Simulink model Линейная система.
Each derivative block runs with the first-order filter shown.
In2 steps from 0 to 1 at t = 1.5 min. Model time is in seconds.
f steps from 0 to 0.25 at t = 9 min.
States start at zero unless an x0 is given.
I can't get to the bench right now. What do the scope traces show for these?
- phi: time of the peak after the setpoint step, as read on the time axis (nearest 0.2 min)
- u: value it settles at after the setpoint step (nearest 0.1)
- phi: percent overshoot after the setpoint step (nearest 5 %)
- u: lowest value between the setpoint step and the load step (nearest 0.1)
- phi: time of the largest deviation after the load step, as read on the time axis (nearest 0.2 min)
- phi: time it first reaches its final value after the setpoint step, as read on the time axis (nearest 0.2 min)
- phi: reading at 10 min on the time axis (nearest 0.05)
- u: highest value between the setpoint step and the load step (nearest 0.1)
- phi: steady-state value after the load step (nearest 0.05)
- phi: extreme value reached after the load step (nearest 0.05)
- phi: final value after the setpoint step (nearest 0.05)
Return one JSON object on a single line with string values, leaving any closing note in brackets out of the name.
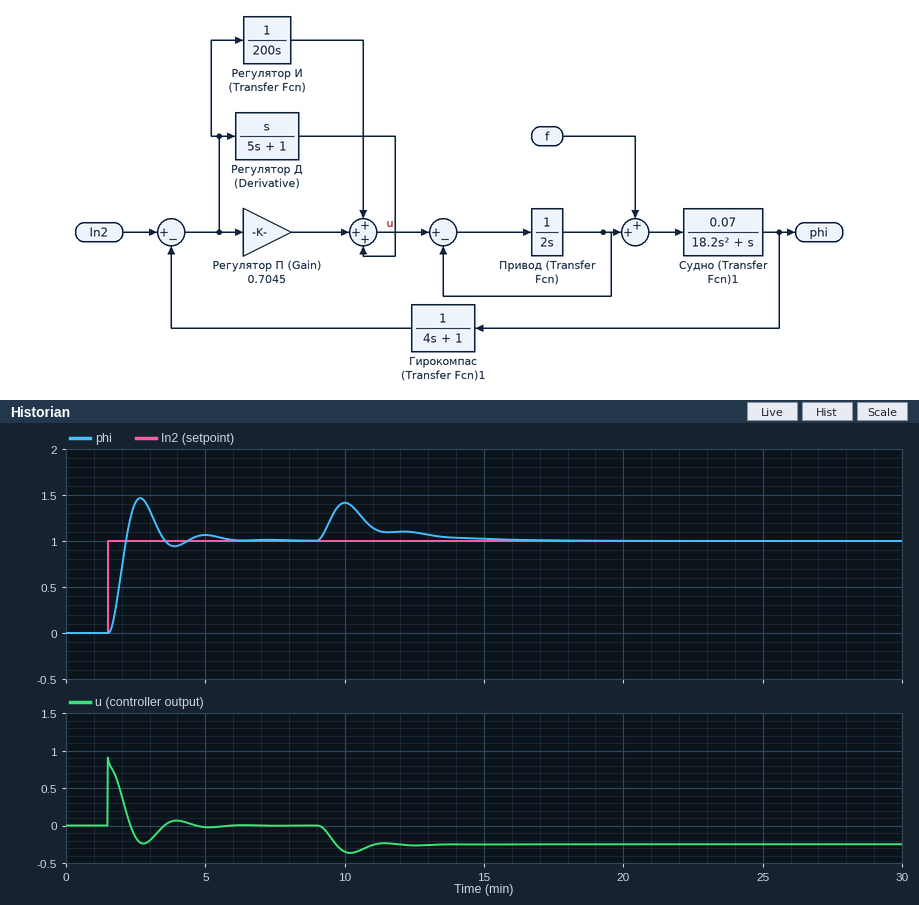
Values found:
{"phi: time of the peak after the setpoint step, as read on the time axis": "2.6 min", "u: value it settles at after the setpoint step": "0.0", "phi: percent overshoot after the setpoint step": "45 %", "u: lowest value between the setpoint step and the load step": "-0.2", "phi: time of the largest deviation after the load step, as read on the time axis": "10.0 min", "phi: time it first reaches its final value after the setpoint step, as read on the time axis": "2.2 min", "phi: reading at 10 min on the time axis": "1.40", "u: highest value between the setpoint step and the load step": "0.9", "phi: steady-state value after the load step": "1.00", "phi: extreme value reached after the load step": "1.40", "phi: final value after the setpoint step": "1.00"}
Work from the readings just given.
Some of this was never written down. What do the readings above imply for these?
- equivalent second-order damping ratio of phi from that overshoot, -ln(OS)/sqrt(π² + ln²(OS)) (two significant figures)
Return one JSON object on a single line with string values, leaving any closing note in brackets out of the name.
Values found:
{"equivalent second-order damping ratio of phi from that overshoot, -ln(OS)/sqrt(π² + ln²(OS))": "0.25"}
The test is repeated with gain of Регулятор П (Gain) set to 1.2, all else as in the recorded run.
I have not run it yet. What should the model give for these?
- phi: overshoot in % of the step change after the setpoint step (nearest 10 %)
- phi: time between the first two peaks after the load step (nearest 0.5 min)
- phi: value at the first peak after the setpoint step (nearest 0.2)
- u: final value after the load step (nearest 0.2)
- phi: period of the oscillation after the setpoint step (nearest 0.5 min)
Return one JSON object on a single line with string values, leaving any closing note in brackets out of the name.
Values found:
{"phi: overshoot in % of the step change after the setpoint step": "60 %", "phi: time between the first two peaks after the load step": "1.5 min", "phi: value at the first peak after the setpoint step": "1.6", "u: final value after the load step": "-0.2", "phi: period of the oscillation after the setpoint step": "1.5 min"}
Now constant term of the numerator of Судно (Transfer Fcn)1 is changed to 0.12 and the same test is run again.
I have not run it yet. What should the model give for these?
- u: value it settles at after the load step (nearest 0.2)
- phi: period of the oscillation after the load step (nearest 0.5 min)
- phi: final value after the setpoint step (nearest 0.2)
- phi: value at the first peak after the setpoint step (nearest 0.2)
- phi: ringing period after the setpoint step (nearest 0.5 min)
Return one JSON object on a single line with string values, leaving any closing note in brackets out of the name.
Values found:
{"u: value it settles at after the load step": "-0.2", "phi: period of the oscillation after the load step": "1.5 min", "phi: final value after the setpoint step": "1.0", "phi: value at the first peak after the setpoint step": "1.6", "phi: ringing period after the setpoint step": "1.5 min"}
